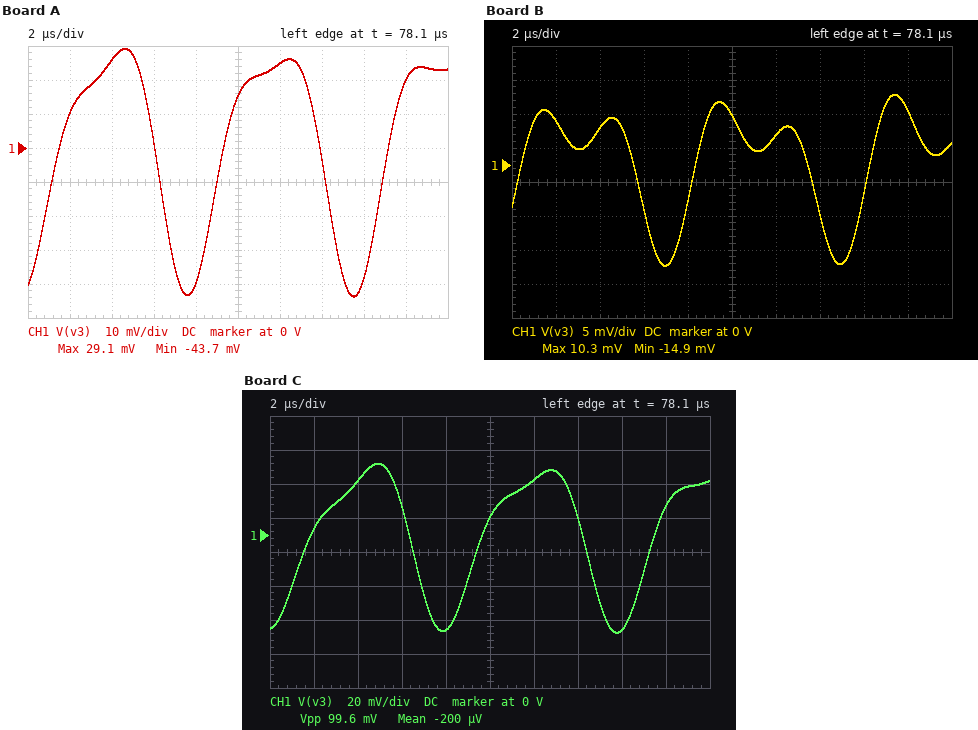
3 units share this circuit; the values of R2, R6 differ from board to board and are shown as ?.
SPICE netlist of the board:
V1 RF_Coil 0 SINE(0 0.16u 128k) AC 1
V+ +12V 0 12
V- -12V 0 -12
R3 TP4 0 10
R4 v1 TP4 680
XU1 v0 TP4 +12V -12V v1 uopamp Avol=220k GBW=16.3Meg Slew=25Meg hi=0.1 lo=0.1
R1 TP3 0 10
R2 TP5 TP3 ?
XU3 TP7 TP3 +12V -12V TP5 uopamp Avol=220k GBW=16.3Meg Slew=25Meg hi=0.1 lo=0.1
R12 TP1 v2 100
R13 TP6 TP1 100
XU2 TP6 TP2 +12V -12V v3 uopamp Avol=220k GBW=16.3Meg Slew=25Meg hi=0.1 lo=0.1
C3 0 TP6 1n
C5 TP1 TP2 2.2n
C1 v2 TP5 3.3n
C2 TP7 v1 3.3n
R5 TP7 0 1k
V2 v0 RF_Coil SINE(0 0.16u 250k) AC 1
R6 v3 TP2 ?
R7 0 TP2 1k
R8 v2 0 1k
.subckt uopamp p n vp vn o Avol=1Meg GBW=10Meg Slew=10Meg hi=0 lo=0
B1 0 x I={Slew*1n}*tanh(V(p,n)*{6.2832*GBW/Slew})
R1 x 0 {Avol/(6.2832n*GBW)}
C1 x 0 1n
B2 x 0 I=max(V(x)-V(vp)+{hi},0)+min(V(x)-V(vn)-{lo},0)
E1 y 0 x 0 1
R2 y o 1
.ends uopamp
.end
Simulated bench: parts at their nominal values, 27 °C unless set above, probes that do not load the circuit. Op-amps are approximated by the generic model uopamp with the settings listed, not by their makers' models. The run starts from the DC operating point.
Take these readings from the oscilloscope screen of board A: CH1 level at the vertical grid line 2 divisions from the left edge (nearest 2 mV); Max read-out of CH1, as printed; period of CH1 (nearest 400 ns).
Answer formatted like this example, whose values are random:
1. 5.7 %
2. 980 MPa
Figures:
1. 26 mV
2. 29.1 mV
3. 8.0 µs
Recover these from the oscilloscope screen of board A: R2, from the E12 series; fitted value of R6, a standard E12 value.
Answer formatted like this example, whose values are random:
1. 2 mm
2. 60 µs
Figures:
1. 820 Ω
2. 39 kΩ
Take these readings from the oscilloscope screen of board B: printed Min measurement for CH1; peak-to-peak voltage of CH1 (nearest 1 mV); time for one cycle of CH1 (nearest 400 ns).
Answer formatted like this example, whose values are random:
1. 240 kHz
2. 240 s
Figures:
1. -14.9 mV
2. 25 mV
3. 8.0 µs
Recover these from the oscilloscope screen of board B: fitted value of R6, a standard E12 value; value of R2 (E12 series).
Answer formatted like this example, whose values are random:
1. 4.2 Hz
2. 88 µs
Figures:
1. 27 kΩ
2. 270 Ω
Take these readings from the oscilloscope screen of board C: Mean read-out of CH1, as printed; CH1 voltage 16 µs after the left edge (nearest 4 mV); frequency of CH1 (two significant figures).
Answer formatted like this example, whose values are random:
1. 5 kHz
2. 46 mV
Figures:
1. -200 µV
2. -56 mV
3. 130 kHz
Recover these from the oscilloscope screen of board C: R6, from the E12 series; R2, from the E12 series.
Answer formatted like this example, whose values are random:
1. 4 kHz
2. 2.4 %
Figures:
1. 33 kΩ
2. 2.2 kΩ
